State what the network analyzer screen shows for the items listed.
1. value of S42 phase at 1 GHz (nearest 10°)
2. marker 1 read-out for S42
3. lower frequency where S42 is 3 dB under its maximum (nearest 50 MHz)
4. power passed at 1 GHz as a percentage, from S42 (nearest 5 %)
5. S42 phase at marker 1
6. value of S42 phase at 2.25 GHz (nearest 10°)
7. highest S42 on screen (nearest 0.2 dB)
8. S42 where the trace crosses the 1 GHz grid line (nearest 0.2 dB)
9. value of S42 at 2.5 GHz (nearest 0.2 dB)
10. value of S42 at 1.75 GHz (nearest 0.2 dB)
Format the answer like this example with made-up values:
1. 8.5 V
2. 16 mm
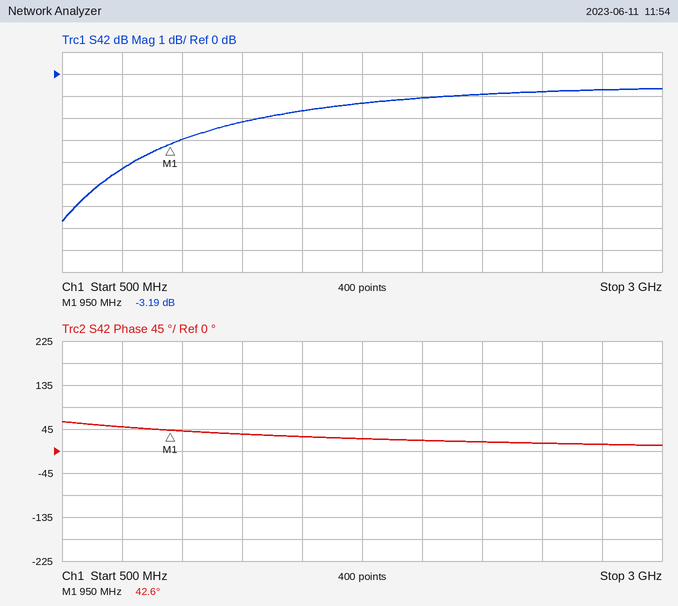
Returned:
1. 40°
2. -3.19 dB
3. 850 MHz
4. 50 %
5. 42.6°
6. 20°
7. -0.6 dB
8. -3.0 dB
9. -0.8 dB
10. -1.4 dB
